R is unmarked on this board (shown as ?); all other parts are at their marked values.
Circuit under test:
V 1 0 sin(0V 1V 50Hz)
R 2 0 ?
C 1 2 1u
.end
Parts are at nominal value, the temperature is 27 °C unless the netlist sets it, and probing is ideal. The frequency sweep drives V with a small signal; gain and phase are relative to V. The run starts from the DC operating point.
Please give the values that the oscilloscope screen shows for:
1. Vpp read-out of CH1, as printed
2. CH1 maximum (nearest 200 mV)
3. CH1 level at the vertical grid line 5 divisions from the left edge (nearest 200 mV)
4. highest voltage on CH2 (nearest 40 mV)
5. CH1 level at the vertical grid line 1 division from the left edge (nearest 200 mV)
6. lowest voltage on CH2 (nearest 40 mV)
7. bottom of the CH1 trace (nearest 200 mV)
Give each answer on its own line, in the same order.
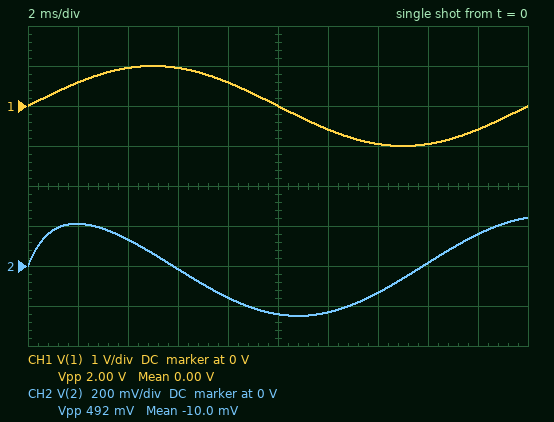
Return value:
2.00 V
1.0 V
0 V
240 mV
600 mV
-240 mV
-1.0 V
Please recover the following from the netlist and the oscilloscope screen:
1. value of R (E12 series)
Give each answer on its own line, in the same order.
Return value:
820 Ω
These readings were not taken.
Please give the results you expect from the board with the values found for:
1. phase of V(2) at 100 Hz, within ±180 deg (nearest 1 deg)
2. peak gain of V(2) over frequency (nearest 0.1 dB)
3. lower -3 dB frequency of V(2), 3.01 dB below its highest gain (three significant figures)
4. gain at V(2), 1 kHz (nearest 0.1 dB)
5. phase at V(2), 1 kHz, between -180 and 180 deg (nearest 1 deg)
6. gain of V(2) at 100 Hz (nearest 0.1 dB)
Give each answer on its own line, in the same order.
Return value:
63 deg
0 dB
194 Hz
-0.2 dB
11 deg
-6.8 dB
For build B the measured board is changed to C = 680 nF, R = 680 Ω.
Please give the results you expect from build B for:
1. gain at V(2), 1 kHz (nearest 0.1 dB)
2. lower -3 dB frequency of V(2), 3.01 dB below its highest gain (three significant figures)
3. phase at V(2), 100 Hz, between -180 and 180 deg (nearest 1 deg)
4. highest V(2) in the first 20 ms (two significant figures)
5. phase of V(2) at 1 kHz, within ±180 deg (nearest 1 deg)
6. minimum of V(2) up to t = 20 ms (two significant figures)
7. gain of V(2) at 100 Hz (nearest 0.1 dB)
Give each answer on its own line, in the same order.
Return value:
-0.5 dB
344 Hz
74 deg
140 mV
19 deg
-140 mV
-11.1 dB
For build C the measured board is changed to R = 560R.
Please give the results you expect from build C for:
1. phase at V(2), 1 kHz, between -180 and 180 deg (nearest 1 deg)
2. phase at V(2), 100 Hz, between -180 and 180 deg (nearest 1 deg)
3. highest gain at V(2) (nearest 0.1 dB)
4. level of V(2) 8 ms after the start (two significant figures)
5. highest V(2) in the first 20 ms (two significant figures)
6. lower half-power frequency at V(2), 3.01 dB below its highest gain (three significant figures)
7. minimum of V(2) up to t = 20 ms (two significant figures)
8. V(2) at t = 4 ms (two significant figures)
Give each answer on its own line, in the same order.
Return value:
16 deg
71 deg
0 dB
-120 mV
170 mV
284 Hz
-170 mV
81 mV
